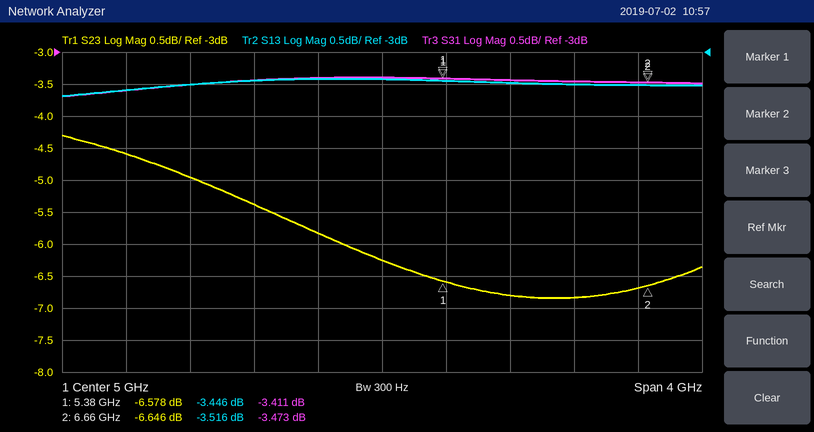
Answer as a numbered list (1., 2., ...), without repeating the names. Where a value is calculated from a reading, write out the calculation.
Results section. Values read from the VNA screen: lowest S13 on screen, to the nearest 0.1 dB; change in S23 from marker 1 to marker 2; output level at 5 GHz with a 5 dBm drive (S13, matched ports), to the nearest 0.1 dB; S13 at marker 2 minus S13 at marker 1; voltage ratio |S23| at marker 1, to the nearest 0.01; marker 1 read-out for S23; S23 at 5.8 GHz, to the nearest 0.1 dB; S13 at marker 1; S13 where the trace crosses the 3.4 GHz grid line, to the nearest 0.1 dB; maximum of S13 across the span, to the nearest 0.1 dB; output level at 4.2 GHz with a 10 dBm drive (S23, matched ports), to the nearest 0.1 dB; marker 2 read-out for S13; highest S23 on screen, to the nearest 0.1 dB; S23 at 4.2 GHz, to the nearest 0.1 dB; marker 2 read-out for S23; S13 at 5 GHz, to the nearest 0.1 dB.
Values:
1. -3.7 dB
2. -6.646 − (-6.578) = -0.068 dB
3. 5 dBm + (-3.4 dB) = 1.6 dBm
4. -3.516 − (-3.446) = -0.070 dB
5. 10^(-6.578/20) ≈ 0.47
6. -6.578 dB
7. -6.8 dB
8. -3.446 dB
9. -3.6 dB
10. -3.4 dB
11. 10 dBm + (-5.4 dB) = 4.6 dBm
12. -3.516 dB
13. -4.3 dB
14. -5.4 dB
15. -6.646 dB
16. -3.4 dB
